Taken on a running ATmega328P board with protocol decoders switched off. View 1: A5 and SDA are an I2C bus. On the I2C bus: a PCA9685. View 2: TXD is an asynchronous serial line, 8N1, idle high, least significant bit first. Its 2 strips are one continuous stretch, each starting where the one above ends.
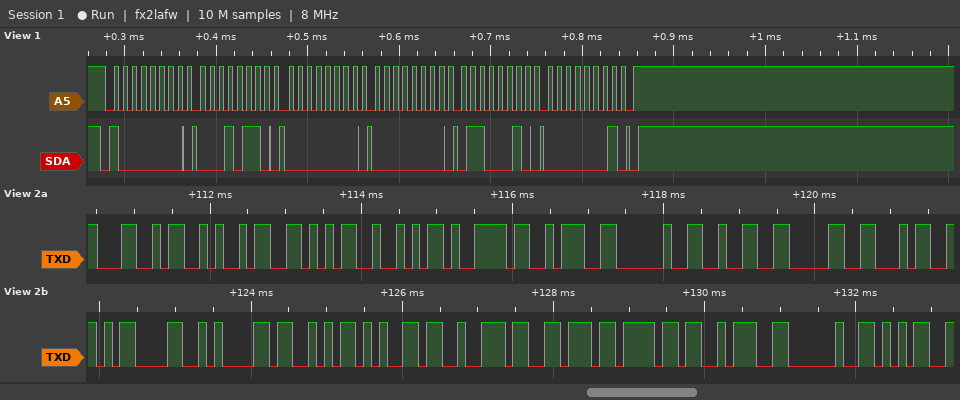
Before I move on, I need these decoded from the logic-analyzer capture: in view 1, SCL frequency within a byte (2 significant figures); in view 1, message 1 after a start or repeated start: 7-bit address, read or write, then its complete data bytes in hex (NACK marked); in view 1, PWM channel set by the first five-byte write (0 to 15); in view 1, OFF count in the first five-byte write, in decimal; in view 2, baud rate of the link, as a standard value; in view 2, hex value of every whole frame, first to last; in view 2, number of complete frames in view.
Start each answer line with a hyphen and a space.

- 100 kHz
- 0x40 write: 16 00 00 62 01
- 4
- 354
- 9600 baud
- 0x4C 0x4A 0x56 0x52 0x79 0x3A 0x20 0x32 0x30 0x34 0x0D 0x0A 0x53 0x65 0x72 0x76 0x6F 0x3A 0x20 0x35
- 20
